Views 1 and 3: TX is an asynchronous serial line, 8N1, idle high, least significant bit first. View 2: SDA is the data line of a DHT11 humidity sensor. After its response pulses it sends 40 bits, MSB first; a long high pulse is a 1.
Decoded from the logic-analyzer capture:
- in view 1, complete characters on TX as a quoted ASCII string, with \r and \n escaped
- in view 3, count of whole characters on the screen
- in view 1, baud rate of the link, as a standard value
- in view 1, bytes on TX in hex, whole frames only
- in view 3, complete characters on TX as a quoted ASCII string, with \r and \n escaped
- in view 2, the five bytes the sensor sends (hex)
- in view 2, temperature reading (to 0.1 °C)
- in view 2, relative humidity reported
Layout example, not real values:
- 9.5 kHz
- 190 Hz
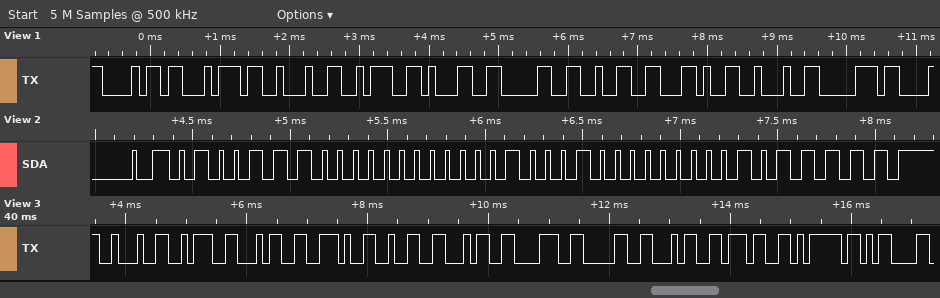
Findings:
- "ht\":102,\"p"
- 12
- 9600 baud
- 68 74 22 3A 31 30 32 2C 22 70
- "\":4.248047}\r"
- 4E 00 11 00 5F
- 17.0 °C
- 78 %
